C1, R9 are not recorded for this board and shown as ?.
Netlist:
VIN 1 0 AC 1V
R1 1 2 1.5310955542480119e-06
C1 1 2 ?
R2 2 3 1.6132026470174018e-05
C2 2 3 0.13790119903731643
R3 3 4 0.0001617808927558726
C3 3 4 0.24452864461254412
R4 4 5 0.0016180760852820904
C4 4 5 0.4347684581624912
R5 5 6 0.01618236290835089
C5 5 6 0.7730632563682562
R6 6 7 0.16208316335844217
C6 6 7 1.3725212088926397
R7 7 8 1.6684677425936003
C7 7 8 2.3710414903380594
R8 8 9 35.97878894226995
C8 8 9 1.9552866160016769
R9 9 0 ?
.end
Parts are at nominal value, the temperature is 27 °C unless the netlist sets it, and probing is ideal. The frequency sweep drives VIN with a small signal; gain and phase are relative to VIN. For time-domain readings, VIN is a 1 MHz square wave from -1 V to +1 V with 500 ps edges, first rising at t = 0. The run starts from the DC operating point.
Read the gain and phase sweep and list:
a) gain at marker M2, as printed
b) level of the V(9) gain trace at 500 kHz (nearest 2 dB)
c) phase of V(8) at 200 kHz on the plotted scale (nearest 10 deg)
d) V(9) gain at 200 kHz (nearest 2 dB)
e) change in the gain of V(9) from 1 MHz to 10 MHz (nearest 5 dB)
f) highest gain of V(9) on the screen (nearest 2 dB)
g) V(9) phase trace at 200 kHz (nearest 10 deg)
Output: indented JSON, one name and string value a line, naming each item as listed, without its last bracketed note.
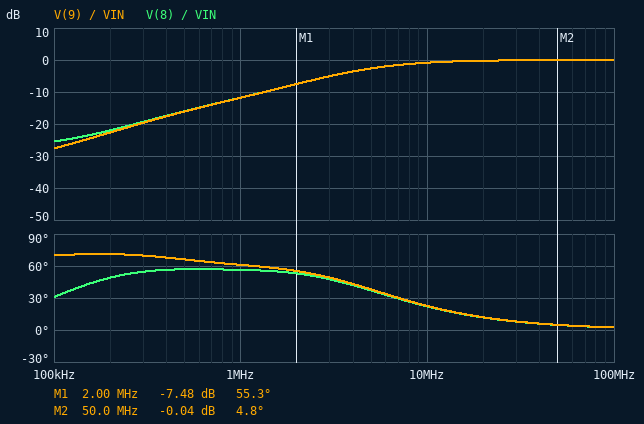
{
  "gain at marker M2, as printed": "-0.04 dB",
  "level of the V(9) gain trace at 500 kHz": "-16 dB",
  "phase of V(8) at 200 kHz on the plotted scale": "50 deg",
  "V(9) gain at 200 kHz": "-22 dB",
  "change in the gain of V(9) from 1 MHz to 10 MHz": "10 dB",
  "highest gain of V(9) on the screen": "0 dB",
  "V(9) phase trace at 200 kHz": "70 deg"
}
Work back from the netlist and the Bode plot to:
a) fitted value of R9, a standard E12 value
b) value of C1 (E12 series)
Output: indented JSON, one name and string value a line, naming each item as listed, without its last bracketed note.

{
  "fitted value of R9, a standard E12 value": "1 µΩ",
  "value of C1": "100 mF"
}
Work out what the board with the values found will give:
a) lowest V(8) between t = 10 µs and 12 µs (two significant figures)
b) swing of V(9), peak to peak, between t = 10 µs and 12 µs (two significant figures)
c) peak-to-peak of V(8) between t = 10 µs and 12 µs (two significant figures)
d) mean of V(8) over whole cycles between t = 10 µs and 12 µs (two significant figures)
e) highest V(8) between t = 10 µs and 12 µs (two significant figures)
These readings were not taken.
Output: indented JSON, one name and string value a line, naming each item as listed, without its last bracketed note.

{
  "lowest V(8) between t = 10 µs and 12 µs": "-2.8 V",
  "swing of V(9), peak to peak, between t = 10 µs and 12 µs": "3.9 V",
  "peak-to-peak of V(8) between t = 10 µs and 12 µs": "3.8 V",
  "mean of V(8) over whole cycles between t = 10 µs and 12 µs": "-890 mV",
  "highest V(8) between t = 10 µs and 12 µs": "1.0 V"
}
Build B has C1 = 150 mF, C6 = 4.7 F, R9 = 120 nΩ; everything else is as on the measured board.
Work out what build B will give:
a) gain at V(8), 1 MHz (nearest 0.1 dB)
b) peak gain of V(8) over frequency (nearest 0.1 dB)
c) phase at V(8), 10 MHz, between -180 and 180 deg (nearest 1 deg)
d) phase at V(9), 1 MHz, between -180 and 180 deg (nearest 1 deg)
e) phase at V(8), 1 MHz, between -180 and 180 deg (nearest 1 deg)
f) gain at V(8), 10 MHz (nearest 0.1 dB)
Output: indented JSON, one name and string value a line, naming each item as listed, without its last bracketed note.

{
  "gain at V(8), 1 MHz": "-27.3 dB",
  "peak gain of V(8) over frequency": "0 dB",
  "phase at V(8), 10 MHz, between -180 and 180 deg": "67 deg",
  "phase at V(9), 1 MHz, between -180 and 180 deg": "78 deg",
  "phase at V(8), 1 MHz, between -180 and 180 deg": "44 deg",
  "gain at V(8), 10 MHz": "-10.1 dB"
}
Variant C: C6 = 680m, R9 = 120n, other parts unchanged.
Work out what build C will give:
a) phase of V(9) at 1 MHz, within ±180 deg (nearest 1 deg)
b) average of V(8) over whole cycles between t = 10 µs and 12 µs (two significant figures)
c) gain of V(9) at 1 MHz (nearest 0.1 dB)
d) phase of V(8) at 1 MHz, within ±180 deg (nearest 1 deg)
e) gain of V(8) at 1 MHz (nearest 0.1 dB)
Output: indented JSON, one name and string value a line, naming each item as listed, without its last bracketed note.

{
  "phase of V(9) at 1 MHz, within ±180 deg": "74 deg",
  "average of V(8) over whole cycles between t = 10 µs and 12 µs": "-900 mV",
  "gain of V(9) at 1 MHz": "-29.7 dB",
  "phase of V(8) at 1 MHz, within ±180 deg": "40 deg",
  "gain of V(8) at 1 MHz": "-28.0 dB"
}
